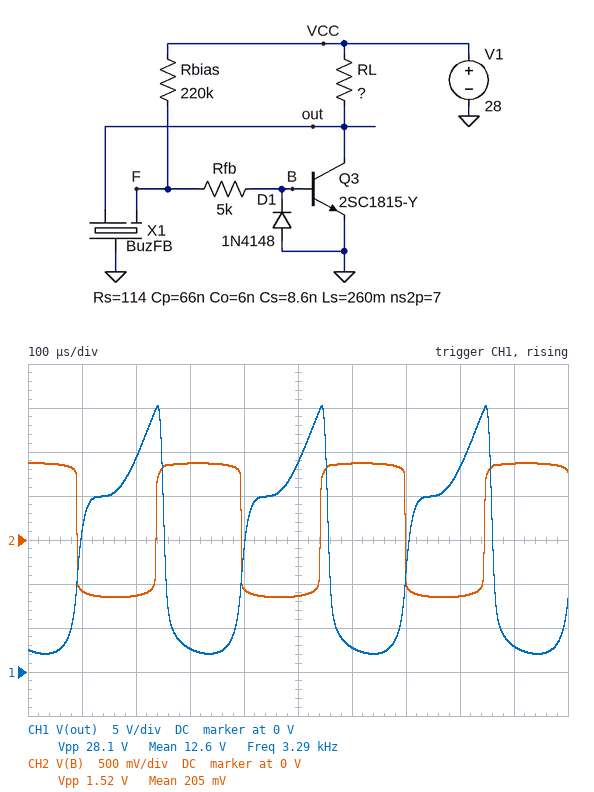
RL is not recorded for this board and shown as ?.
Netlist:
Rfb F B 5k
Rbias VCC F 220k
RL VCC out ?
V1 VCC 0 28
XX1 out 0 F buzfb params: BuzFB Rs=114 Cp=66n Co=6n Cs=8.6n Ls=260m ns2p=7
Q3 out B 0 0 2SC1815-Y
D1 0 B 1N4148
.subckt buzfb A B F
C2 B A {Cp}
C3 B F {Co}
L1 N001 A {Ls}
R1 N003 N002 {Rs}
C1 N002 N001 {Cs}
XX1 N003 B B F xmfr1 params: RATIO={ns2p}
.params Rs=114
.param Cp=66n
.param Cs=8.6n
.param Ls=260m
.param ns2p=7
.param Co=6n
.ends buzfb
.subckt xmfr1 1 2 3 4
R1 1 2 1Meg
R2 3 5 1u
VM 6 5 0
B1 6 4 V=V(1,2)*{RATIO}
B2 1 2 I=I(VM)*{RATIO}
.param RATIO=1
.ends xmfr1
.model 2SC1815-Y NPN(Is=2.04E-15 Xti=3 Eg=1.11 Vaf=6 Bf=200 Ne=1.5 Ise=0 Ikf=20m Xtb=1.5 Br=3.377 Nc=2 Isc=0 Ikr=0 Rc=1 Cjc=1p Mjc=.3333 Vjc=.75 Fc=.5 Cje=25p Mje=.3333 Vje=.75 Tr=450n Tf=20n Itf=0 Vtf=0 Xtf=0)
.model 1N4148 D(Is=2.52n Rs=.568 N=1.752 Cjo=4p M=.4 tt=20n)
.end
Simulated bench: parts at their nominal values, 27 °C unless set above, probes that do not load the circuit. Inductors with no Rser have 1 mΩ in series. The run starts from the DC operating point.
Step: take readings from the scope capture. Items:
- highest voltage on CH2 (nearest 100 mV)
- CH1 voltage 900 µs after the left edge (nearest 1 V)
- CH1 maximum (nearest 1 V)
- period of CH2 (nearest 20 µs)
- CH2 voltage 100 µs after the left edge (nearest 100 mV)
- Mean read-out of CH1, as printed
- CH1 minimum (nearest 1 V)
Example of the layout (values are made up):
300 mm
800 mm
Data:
900 mV
3 V
30 V
300 µs
-600 mV
12.6 V
2 V
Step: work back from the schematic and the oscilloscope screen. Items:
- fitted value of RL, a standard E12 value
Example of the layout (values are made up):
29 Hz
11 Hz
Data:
220 Ω
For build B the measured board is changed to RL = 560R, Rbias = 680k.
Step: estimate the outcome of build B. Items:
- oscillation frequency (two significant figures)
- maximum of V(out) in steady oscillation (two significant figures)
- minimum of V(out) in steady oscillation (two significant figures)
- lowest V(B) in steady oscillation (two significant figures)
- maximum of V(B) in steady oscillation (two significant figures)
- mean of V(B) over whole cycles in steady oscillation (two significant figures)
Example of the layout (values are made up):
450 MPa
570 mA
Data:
3.2 kHz
28 V
180 mV
-630 mV
850 mV
130 mV
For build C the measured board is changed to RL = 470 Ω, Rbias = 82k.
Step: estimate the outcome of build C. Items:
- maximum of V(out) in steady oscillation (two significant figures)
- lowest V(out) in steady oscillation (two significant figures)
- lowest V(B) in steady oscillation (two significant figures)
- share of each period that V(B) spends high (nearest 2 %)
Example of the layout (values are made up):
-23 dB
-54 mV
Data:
27 V
200 mV
-630 mV
54 %
